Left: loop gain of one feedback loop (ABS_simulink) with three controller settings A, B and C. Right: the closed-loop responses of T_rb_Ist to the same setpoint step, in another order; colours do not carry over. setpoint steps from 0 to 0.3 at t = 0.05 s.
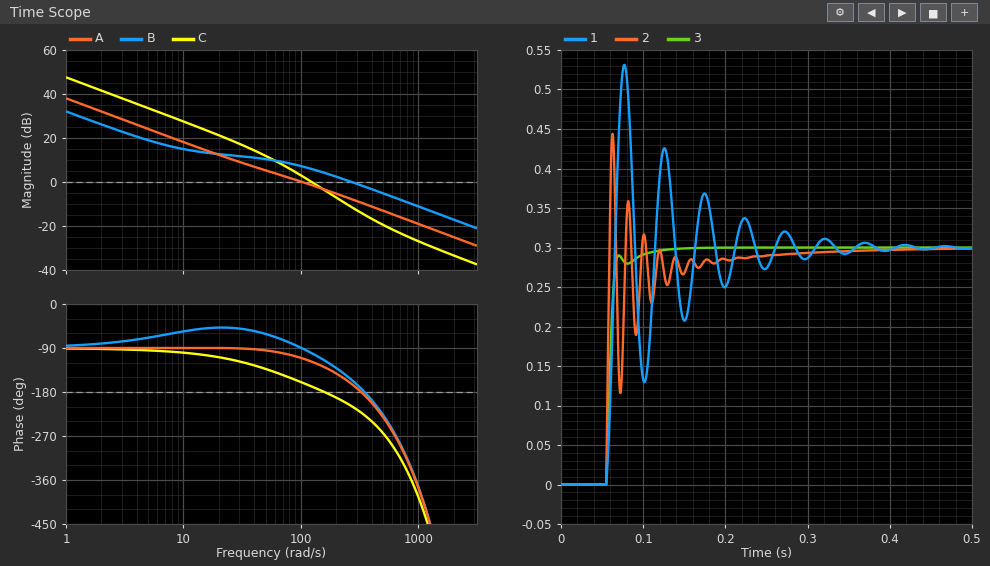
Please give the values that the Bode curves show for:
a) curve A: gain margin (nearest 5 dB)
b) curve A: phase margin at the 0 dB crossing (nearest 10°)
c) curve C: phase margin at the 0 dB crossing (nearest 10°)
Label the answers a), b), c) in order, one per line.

a) 10 dB
b) 70°
c) 10°
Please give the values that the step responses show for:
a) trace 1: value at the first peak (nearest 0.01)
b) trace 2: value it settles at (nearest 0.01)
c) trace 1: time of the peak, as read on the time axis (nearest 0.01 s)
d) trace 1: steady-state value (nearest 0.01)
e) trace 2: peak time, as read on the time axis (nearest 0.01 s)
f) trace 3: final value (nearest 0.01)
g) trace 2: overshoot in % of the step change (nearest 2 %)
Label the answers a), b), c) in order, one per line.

a) 0.53
b) 0.30
c) 0.08 s
d) 0.30
e) 0.06 s
f) 0.30
g) 48 %
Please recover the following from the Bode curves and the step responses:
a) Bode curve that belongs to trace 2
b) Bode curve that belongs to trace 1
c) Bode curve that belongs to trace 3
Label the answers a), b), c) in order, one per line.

a) B
b) C
c) A
